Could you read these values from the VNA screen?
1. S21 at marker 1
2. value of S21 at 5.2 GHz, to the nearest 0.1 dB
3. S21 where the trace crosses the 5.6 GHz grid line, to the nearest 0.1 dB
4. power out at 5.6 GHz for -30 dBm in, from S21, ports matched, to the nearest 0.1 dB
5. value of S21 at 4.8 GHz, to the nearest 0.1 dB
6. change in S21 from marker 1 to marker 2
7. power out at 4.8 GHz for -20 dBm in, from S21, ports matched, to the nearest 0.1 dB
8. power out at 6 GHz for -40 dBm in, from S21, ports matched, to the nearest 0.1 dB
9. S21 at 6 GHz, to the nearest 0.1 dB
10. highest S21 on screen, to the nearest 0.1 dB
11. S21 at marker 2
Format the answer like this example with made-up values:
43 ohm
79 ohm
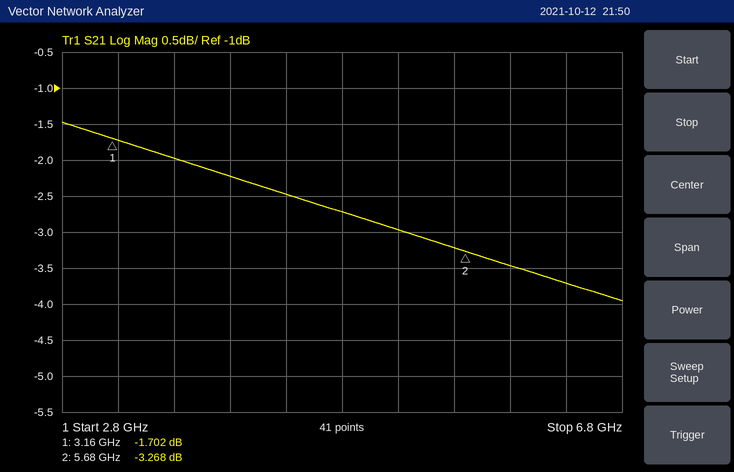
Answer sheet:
-1.702 dB
-3.0 dB
-3.2 dB
-33.2 dBm
-2.7 dB
-1.566 dB
-22.7 dBm
-43.5 dBm
-3.5 dB
-1.5 dB
-3.268 dB
